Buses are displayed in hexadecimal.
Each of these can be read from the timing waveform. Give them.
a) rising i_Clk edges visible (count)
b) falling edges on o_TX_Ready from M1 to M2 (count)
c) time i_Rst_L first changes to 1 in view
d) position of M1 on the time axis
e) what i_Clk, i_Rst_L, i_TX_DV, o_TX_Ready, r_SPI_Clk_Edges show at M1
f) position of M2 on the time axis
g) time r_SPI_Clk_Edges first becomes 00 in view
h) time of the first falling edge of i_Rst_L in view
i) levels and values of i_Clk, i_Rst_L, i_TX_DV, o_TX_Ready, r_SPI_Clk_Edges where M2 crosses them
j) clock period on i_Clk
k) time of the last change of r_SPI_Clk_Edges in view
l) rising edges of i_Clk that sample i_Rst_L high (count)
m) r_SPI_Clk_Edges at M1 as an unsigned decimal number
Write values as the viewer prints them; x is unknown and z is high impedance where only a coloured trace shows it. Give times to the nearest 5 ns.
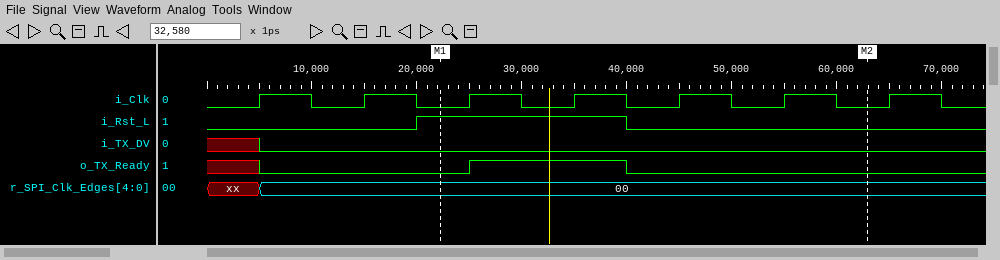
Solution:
7
1
20 ns
20 ns
i_Clk=0, i_Rst_L=1, i_TX_DV=0, o_TX_Ready=0, r_SPI_Clk_Edges=00
65 ns
5 ns
40 ns
i_Clk=0, i_Rst_L=0, i_TX_DV=0, o_TX_Ready=0, r_SPI_Clk_Edges=00
10 ns
5 ns
2
0
